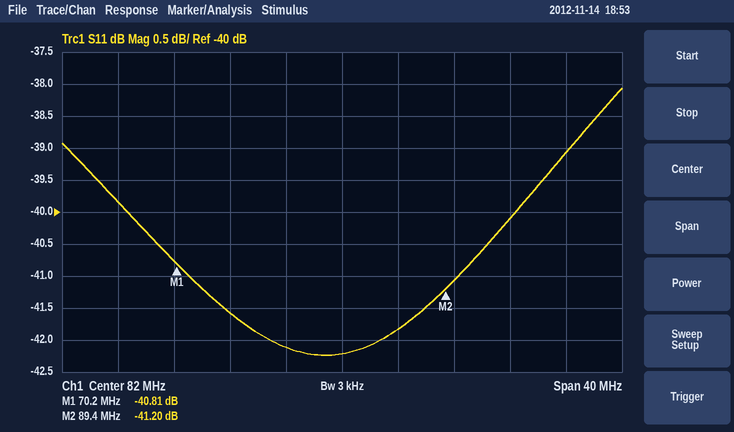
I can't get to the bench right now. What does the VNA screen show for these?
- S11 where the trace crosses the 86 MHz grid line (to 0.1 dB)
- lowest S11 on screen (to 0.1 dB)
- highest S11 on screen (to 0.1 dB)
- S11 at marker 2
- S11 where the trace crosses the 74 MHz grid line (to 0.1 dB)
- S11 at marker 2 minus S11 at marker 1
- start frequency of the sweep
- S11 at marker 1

-41.8 dB
-42.2 dB
-38.1 dB
-41.20 dB
-41.6 dB
-0.39 dB
62 MHz
-40.81 dB
